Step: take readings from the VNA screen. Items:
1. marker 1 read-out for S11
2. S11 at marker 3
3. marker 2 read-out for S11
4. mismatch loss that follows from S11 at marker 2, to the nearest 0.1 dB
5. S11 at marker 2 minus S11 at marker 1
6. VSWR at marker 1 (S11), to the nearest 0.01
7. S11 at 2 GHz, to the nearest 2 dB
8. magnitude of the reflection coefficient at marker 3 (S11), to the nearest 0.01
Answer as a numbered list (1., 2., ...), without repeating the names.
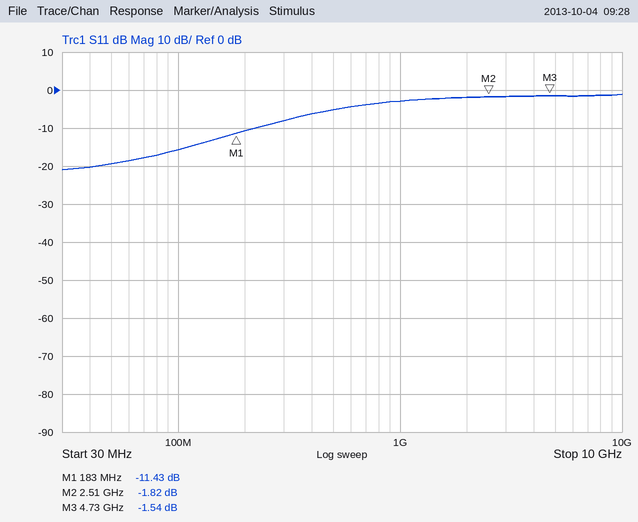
1. -11.43 dB
2. -1.54 dB
3. -1.82 dB
4. 4.7 dB
5. 9.61 dB
6. 1.73
7. -2 dB
8. 0.84
